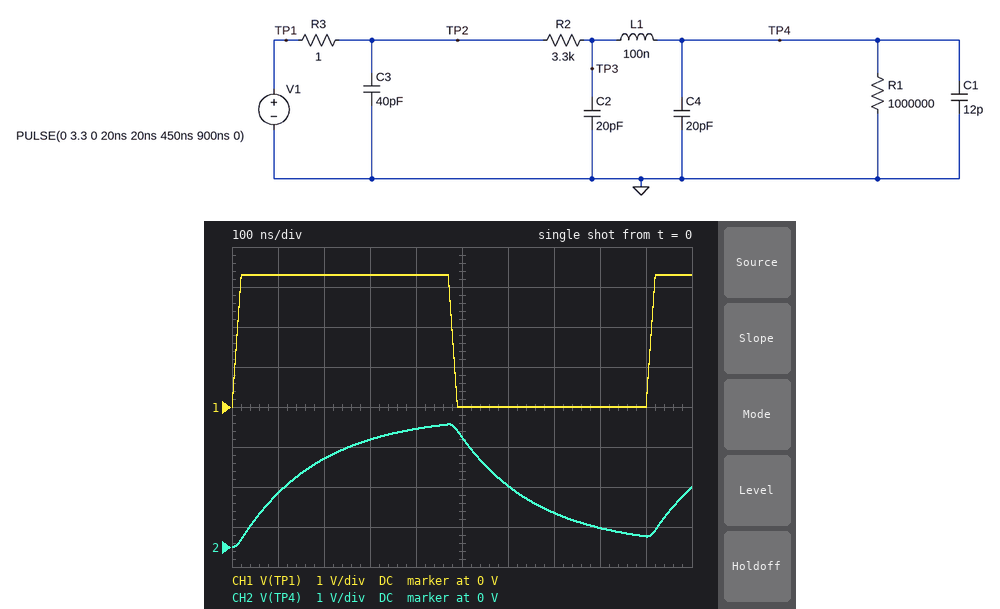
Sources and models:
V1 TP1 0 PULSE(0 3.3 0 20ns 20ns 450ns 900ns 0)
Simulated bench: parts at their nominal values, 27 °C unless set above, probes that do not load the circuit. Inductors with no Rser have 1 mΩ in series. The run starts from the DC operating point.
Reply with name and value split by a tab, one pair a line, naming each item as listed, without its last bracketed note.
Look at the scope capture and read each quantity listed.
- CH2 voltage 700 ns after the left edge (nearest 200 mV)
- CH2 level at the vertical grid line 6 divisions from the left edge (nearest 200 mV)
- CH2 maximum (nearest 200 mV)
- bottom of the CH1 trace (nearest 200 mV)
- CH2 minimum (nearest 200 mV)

CH2 voltage 700 ns after the left edge	800 mV
CH2 level at the vertical grid line 6 divisions from the left edge	1.6 V
CH2 maximum	3.0 V
bottom of the CH1 trace	0 V
CH2 minimum	0 V
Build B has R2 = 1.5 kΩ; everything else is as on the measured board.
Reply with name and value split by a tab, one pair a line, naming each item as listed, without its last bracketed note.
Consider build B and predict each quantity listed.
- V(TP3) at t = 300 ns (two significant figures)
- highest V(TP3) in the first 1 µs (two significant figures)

V(TP3) at t = 300 ns	3.2 V
highest V(TP3) in the first 1 µs	3.3 V
